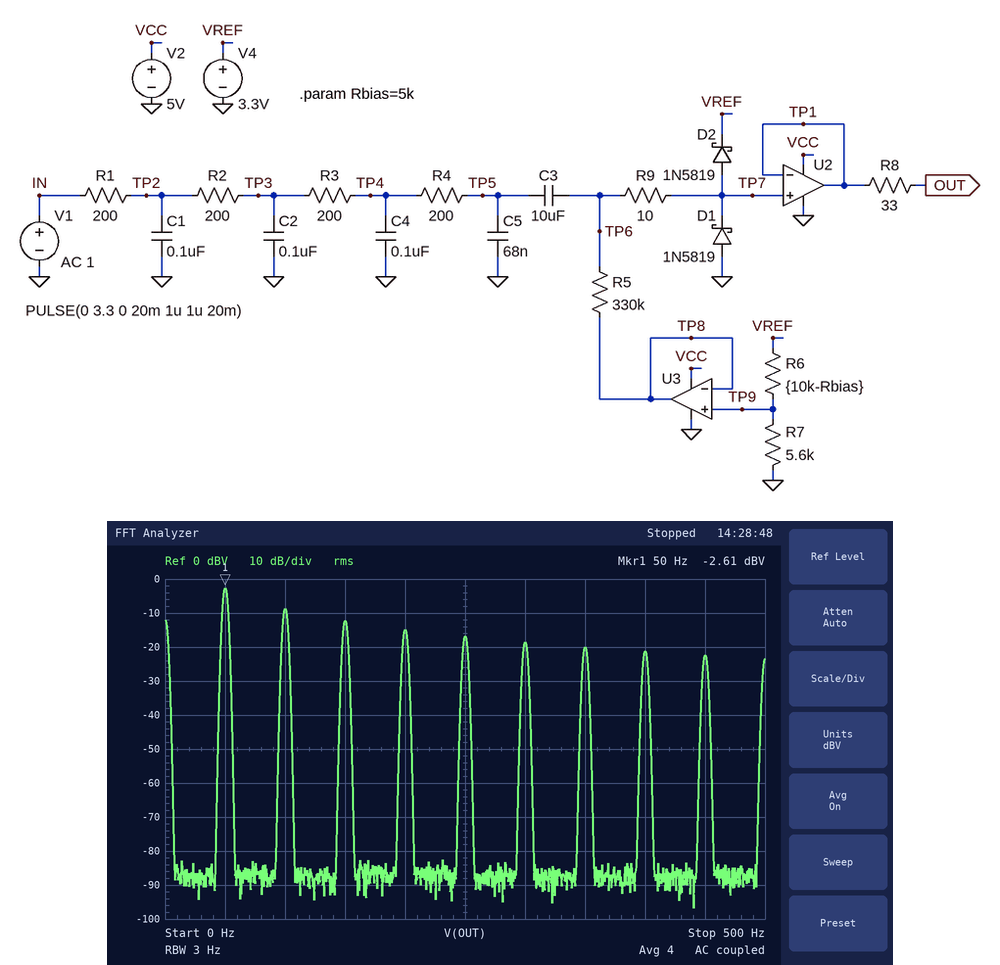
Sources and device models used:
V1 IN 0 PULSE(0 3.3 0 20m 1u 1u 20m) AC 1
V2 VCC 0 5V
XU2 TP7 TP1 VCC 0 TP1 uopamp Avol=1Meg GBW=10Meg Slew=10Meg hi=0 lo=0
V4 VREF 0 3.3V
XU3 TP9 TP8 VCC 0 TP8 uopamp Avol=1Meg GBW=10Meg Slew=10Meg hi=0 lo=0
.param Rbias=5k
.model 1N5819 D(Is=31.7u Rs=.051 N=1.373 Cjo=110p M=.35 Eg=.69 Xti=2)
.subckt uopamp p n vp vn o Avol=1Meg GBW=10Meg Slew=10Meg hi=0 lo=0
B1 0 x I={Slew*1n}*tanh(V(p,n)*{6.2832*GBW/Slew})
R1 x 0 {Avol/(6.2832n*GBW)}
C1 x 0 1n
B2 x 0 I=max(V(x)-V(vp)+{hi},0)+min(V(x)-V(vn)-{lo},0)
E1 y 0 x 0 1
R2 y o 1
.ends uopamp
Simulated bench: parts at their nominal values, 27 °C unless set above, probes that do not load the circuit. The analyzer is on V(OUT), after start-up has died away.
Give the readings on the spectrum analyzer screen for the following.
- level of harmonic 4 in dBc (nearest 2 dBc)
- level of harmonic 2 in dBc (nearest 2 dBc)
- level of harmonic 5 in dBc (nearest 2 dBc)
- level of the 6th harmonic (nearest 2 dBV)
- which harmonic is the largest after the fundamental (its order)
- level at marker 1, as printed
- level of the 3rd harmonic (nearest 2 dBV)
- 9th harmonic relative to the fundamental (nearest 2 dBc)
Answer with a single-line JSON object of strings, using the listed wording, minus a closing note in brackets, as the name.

{"level of harmonic 4 in dBc": "-12 dBc", "level of harmonic 2 in dBc": "-6 dBc", "level of harmonic 5 in dBc": "-14 dBc", "level of the 6th harmonic": "-18 dBV", "which harmonic is the largest after the fundamental": "2", "level at marker 1, as printed": "-2.61 dBV", "level of the 3rd harmonic": "-12 dBV", "9th harmonic relative to the fundamental": "-20 dBc"}
